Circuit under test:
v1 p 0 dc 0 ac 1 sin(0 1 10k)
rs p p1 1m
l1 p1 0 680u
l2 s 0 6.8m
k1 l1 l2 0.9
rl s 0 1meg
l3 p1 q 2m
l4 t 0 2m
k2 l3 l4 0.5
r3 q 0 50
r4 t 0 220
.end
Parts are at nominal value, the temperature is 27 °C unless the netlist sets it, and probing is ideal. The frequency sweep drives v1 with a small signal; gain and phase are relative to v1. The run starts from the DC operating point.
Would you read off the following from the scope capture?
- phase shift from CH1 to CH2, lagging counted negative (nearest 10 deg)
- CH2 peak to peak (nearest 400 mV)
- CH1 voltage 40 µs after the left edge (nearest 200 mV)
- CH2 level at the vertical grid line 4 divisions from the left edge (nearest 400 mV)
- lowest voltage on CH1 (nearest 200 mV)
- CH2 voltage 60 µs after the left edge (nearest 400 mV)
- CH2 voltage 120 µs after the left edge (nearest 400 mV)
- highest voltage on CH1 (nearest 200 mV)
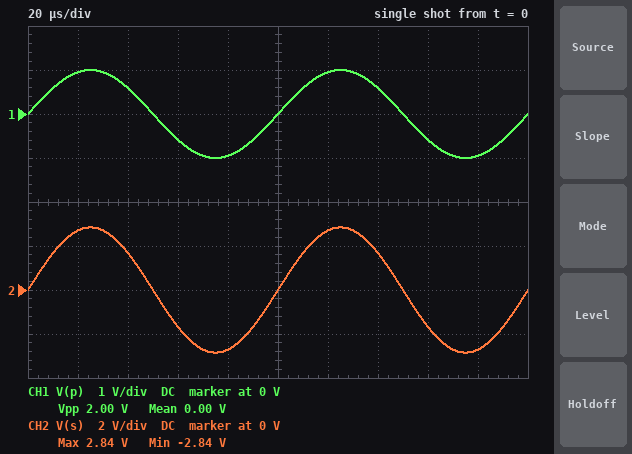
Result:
0 deg
5.6 V
600 mV
-2.8 V
-1.0 V
-1.6 V
2.8 V
1.0 V
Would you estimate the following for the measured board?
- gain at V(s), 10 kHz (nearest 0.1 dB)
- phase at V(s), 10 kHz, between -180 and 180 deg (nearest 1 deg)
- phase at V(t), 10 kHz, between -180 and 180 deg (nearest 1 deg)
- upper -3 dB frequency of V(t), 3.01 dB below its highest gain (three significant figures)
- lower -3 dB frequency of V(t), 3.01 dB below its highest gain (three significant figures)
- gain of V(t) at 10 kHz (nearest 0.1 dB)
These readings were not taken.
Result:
9.1 dB
0 deg
-1 deg
31.6 kHz
2.94 kHz
-7.8 dB
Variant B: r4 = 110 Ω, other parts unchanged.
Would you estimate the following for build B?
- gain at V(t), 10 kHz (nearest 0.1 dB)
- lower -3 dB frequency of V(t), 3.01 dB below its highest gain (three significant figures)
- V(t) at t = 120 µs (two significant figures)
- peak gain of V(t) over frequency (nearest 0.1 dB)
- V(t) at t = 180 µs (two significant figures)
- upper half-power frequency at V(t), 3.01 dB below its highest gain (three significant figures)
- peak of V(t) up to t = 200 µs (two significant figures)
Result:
-9.7 dB
2.40 kHz
250 mV
-9.3 dB
-330 mV
19.4 kHz
320 mV
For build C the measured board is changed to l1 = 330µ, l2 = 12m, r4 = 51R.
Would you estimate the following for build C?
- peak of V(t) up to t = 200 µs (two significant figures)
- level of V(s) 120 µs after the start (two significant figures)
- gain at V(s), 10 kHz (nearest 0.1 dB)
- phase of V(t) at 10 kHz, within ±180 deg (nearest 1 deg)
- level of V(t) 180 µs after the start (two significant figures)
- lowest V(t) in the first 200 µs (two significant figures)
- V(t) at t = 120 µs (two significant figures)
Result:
190 mV
5.2 V
14.7 dB
-36 deg
-200 mV
-230 mV
100 mV
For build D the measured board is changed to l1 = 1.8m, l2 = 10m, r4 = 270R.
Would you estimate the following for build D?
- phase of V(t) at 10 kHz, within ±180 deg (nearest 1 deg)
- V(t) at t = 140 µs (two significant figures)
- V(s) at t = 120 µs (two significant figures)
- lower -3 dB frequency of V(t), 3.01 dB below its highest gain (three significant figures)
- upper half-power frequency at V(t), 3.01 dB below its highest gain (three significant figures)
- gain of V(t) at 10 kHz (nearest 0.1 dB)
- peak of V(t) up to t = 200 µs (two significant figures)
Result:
2 deg
230 mV
2.0 V
3.08 kHz
37.0 kHz
-7.5 dB
410 mV
